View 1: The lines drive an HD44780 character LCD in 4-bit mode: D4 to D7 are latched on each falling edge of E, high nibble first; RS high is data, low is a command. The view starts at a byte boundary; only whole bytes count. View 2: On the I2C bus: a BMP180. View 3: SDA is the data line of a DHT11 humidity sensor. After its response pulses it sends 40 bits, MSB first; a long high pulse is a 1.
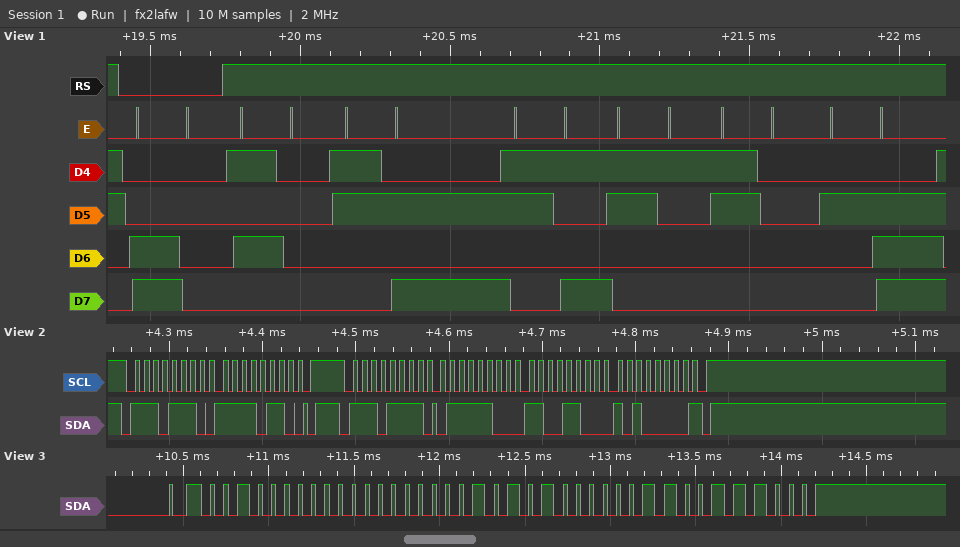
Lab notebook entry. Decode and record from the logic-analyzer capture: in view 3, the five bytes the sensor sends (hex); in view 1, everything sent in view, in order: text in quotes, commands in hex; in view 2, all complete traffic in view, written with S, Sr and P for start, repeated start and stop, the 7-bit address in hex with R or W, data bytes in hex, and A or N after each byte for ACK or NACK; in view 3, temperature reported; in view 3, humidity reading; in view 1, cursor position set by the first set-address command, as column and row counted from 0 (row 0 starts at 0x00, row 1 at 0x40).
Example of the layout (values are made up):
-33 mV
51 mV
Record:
20 00 15 03 38
0xC0 "P:910."
S 77W A F6 A P S 77R A 7C A CC A A0 N P
21.3 °C
32 %
column 0, row 1
